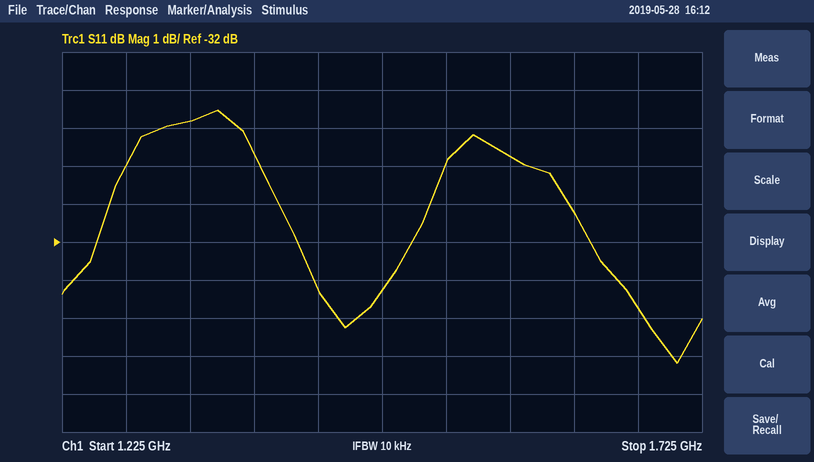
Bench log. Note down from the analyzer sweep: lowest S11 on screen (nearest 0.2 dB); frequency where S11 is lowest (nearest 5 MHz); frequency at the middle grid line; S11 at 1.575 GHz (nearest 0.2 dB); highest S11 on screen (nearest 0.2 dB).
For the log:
-35.2 dB
1.705 GHz
1.475 GHz
-29.8 dB
-28.6 dB
